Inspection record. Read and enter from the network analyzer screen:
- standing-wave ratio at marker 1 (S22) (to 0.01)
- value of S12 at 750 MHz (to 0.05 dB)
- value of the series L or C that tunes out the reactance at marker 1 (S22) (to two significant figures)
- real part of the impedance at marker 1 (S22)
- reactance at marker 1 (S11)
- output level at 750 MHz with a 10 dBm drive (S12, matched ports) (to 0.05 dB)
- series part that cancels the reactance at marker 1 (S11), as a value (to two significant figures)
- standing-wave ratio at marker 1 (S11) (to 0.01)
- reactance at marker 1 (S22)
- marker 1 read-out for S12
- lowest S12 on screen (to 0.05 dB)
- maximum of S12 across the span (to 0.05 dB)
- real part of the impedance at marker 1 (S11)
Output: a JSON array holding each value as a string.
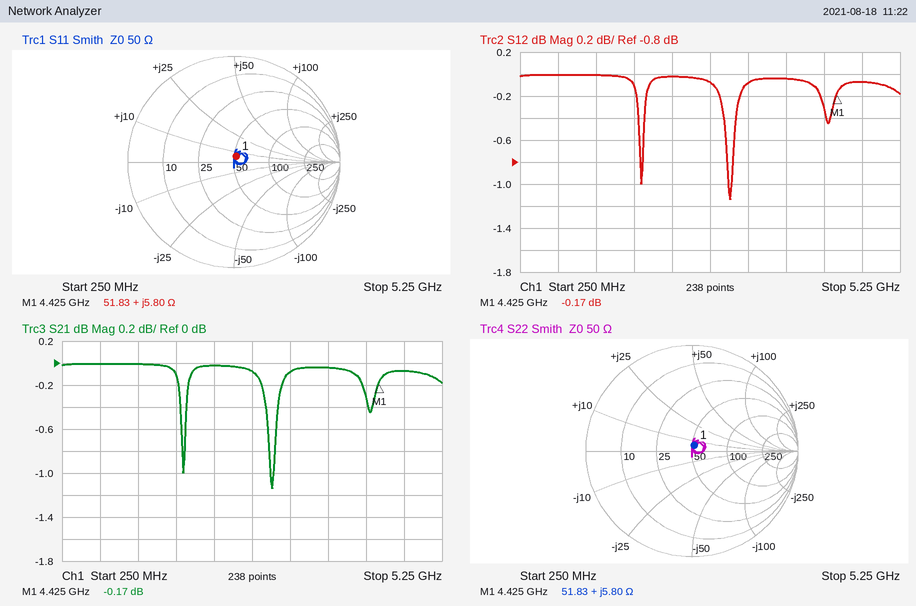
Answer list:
["1.13", "0.00 dB", "6.2 pF", "51.83 Ω", "+5.80 Ω", "10.00 dBm", "6.2 pF", "1.13", "+5.80 Ω", "-0.17 dB", "-1.15 dB", "0.00 dB", "51.83 Ω"]
